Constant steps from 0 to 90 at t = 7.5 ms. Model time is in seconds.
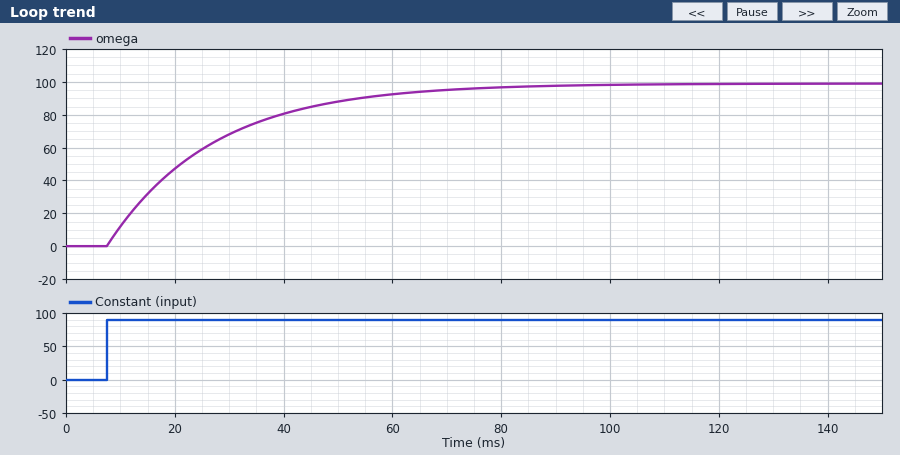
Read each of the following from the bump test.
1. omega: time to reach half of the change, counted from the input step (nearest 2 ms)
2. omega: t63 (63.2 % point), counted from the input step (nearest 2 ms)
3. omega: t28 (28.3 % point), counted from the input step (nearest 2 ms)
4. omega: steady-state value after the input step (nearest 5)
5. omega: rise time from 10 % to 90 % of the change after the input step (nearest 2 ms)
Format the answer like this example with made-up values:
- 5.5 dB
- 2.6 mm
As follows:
- 14 ms
- 20 ms
- 6 ms
- 100
- 42 ms
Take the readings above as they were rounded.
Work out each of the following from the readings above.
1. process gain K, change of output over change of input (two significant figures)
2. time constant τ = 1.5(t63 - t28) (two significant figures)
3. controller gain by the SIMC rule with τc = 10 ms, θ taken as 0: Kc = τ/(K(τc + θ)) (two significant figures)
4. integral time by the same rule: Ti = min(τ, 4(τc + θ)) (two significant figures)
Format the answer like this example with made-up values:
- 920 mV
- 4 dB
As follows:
- 1.1
- 21 ms
- 1.9
- 21 ms
